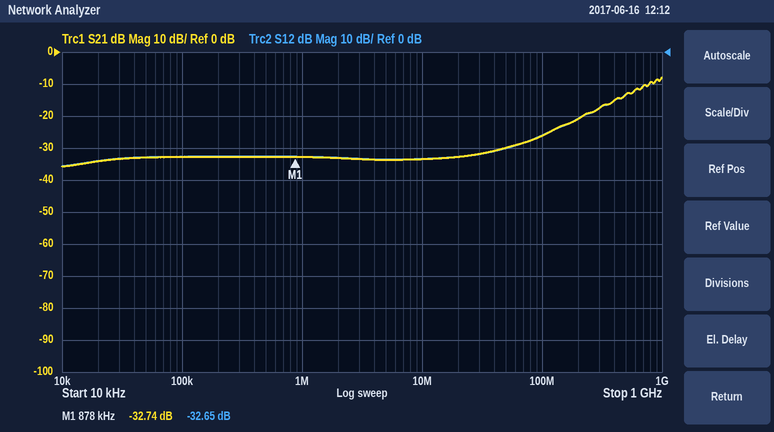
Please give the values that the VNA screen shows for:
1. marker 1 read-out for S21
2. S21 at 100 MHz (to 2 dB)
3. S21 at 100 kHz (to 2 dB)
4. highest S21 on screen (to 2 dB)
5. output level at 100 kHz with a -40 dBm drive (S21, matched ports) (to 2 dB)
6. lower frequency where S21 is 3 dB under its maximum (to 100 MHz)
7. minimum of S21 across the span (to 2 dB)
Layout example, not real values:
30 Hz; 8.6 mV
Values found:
-32.74 dB; -26 dB; -32 dB; -8 dB; -72 dBm; 700 MHz; -36 dB
